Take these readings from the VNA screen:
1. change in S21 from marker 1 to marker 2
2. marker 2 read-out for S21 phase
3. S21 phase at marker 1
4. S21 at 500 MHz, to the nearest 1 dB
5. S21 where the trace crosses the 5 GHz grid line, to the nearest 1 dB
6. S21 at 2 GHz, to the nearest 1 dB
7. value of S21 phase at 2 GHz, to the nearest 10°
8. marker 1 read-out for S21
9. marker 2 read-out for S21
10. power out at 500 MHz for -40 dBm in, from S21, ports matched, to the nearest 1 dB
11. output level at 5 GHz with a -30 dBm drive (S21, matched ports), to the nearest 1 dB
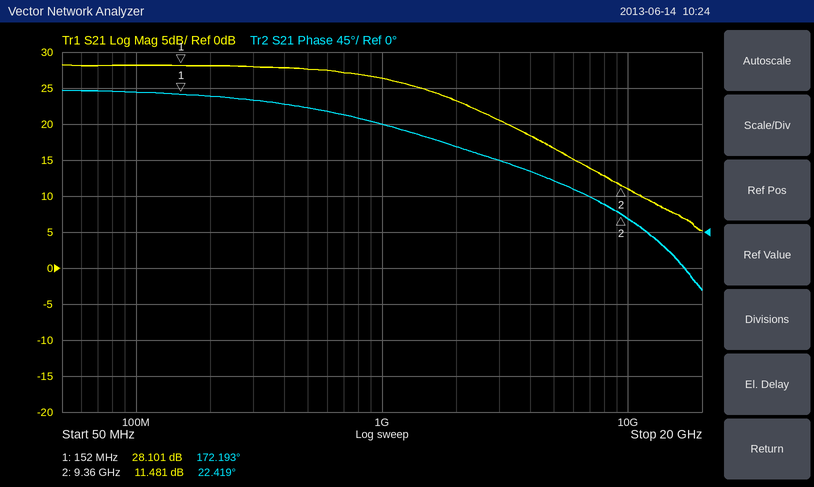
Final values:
-16.620 dB
22.419°
172.193°
28 dB
17 dB
23 dB
110°
28.101 dB
11.481 dB
-12 dBm
-13 dBm
